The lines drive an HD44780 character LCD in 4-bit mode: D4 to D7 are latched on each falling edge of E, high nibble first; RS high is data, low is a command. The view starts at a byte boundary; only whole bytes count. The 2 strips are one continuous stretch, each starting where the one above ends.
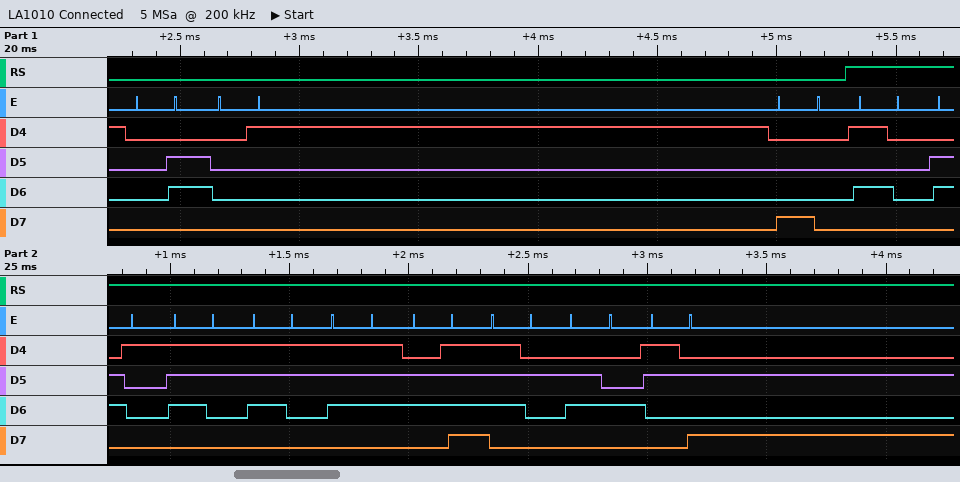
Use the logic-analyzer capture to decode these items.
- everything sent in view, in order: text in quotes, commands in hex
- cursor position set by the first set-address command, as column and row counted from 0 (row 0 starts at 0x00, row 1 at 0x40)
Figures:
0x06 0x01 0x80 "Password:"
column 0, row 0
